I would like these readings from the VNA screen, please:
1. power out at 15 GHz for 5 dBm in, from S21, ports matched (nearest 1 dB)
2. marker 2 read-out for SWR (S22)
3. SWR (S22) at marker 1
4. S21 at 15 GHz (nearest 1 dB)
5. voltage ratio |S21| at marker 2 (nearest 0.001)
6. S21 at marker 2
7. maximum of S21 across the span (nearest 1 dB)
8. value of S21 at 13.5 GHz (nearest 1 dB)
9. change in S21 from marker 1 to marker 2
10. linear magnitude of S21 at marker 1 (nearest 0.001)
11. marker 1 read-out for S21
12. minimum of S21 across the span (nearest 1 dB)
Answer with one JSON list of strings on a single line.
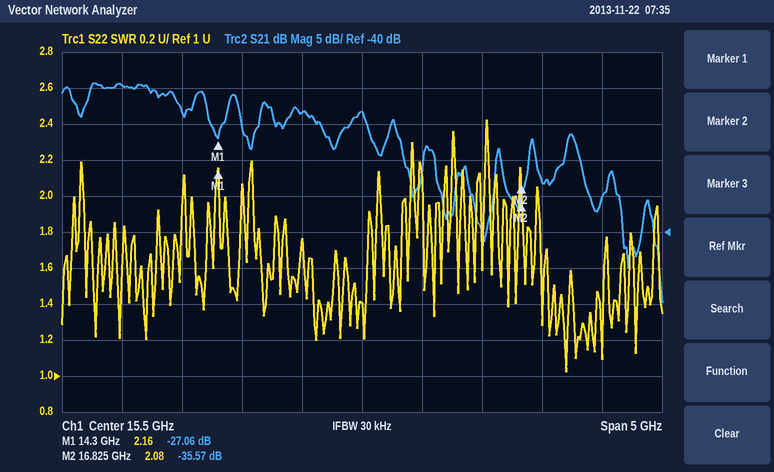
["-18 dBm", "2.08", "2.16", "-23 dB", "0.017", "-35.57 dB", "-19 dB", "-20 dB", "-8.51 dB", "0.044", "-27.06 dB", "-50 dB"]
